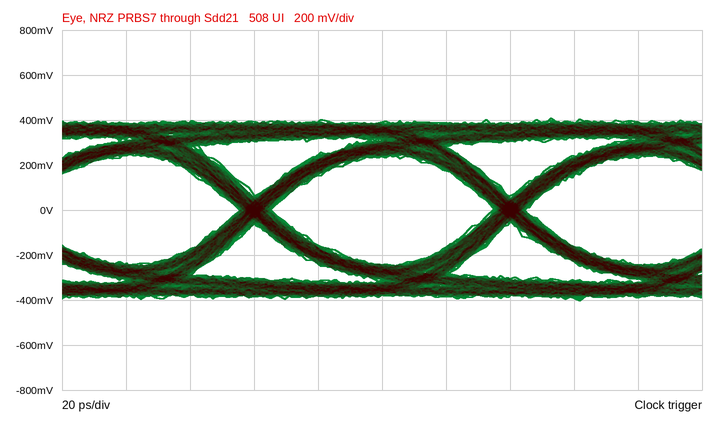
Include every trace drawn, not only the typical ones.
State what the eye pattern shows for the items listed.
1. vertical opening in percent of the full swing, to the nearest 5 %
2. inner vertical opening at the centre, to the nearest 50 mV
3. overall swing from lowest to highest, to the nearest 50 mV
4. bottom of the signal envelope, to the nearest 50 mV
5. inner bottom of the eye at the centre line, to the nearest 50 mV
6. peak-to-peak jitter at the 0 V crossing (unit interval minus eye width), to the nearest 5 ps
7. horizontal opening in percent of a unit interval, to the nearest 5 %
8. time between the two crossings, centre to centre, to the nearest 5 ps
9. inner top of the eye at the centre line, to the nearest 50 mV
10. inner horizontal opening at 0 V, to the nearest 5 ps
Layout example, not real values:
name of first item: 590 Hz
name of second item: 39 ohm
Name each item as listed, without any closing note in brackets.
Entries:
vertical opening in percent of the full swing, to the nearest 5 %: 60 %
inner vertical opening at the centre, to the nearest 50 mV: 500 mV
overall swing from lowest to highest, to the nearest 50 mV: 800 mV
bottom of the signal envelope, to the nearest 50 mV: -400 mV
inner bottom of the eye at the centre line, to the nearest 50 mV: -250 mV
peak-to-peak jitter at the 0 V crossing (unit interval minus eye width), to the nearest 5 ps: 10 ps
horizontal opening in percent of a unit interval, to the nearest 5 %: 85 %
time between the two crossings, centre to centre, to the nearest 5 ps: 80 ps
inner top of the eye at the centre line, to the nearest 50 mV: 250 mV
inner horizontal opening at 0 V, to the nearest 5 ps: 70 ps
